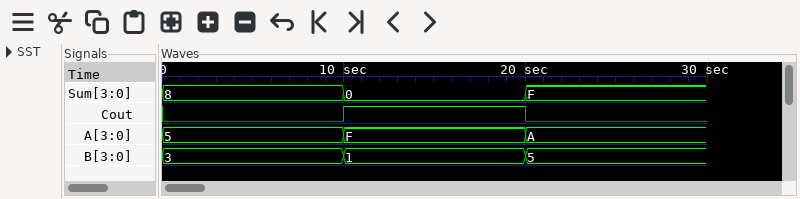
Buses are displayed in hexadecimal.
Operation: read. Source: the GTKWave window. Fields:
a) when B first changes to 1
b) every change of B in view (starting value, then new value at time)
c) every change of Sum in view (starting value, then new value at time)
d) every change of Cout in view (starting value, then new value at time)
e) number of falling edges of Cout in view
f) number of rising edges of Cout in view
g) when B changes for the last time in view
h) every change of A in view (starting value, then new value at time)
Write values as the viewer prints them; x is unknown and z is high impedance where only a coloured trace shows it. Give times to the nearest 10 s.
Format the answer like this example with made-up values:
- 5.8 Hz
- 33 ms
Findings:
- 10 s
- 3, 1 at 10 s, 5 at 20 s
- 8, 0 at 10 s, F at 20 s
- 0, 1 at 10 s, 0 at 20 s
- 1
- 1
- 20 s
- 5, F at 10 s, A at 20 s
